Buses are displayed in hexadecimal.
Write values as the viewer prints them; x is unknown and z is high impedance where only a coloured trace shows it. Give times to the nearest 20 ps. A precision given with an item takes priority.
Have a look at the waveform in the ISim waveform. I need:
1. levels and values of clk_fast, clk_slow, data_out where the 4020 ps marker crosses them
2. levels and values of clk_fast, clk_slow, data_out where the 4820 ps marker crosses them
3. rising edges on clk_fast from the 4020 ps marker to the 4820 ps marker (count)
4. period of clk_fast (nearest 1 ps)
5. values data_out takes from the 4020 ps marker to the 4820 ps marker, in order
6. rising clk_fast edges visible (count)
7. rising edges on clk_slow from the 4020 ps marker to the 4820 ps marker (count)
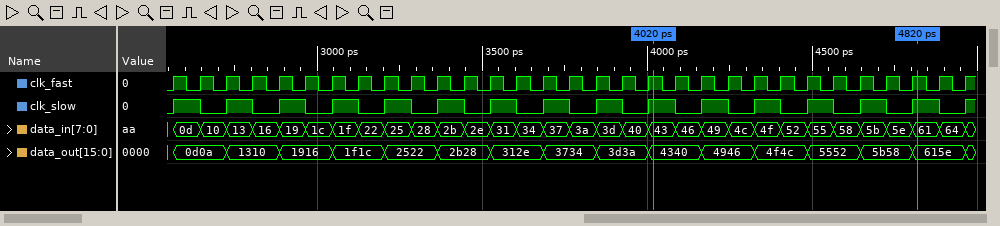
clk_fast=1, clk_slow=1, data_out=4340
clk_fast=1, clk_slow=1, data_out=615e
10
80 ps
4340, 4946, 4f4c, 5552, 5b58, 615e
31
5
